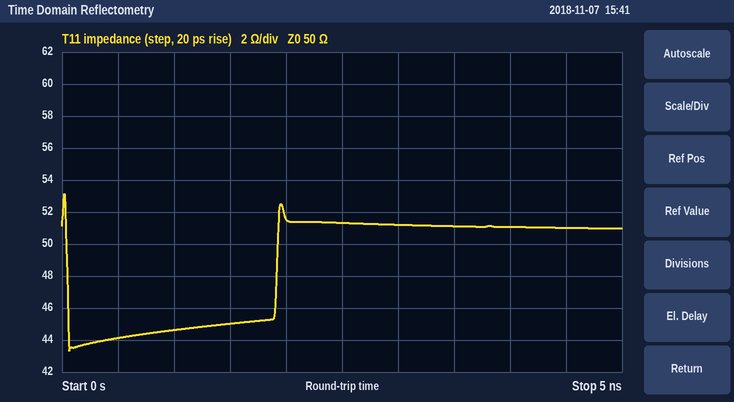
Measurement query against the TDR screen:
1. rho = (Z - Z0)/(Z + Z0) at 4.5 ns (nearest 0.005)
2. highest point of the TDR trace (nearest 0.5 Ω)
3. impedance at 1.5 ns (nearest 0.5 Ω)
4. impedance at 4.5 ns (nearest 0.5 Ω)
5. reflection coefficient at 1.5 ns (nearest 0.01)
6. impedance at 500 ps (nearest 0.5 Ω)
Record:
+0.010
53.0 Ω
45.0 Ω
51.0 Ω
-0.05
44.0 Ω
